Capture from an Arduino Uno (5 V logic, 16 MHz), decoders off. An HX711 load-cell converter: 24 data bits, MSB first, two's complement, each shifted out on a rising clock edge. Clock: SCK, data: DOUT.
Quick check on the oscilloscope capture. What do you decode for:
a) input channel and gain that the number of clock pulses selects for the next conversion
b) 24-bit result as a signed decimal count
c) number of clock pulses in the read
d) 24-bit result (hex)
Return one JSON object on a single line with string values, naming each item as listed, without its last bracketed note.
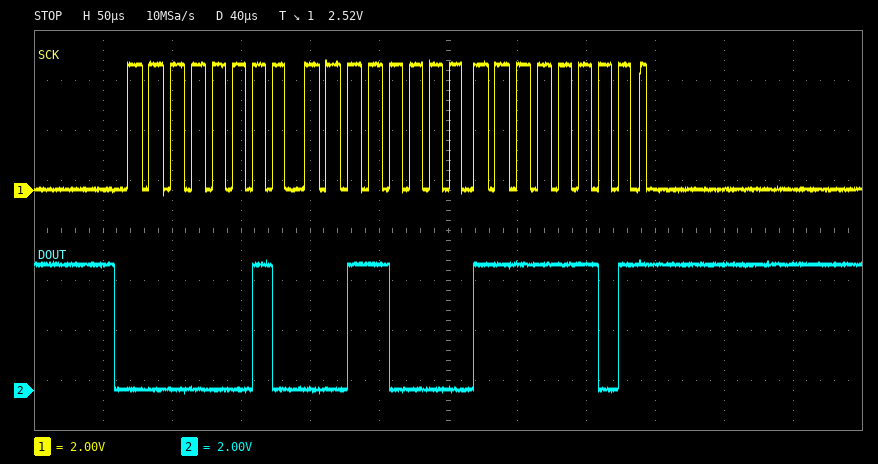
{"input channel and gain that the number of clock pulses selects for the next conversion": "channel A, gain 128", "24-bit result as a signed decimal count": "143613", "number of clock pulses in the read": "25", "24-bit result": "0x0230FD"}
